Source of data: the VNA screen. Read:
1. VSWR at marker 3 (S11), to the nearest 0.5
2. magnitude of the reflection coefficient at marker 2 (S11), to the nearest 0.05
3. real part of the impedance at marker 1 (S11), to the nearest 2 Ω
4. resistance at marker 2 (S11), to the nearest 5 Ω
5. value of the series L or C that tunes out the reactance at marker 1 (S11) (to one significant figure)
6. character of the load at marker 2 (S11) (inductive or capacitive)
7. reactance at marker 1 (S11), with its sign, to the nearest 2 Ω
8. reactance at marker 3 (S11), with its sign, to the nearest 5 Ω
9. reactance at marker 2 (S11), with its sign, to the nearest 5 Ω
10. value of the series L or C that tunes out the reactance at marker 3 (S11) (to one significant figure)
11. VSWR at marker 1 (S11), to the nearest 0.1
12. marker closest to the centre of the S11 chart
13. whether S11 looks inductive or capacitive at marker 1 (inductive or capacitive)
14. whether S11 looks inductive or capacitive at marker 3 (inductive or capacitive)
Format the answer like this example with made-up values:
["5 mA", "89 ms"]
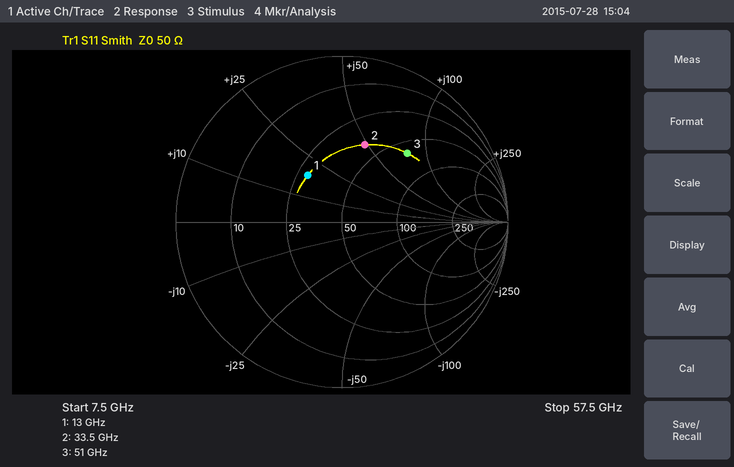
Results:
["3.5", "0.50", "28 Ω", "40 Ω", "700 fF", "inductive", "+18 Ω", "+75 Ω", "+50 Ω", "40 fF", "2.1", "marker 1", "inductive", "inductive"]
